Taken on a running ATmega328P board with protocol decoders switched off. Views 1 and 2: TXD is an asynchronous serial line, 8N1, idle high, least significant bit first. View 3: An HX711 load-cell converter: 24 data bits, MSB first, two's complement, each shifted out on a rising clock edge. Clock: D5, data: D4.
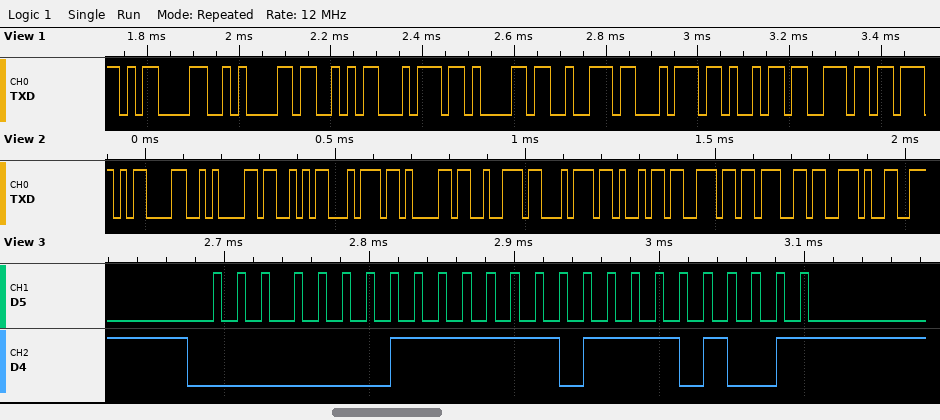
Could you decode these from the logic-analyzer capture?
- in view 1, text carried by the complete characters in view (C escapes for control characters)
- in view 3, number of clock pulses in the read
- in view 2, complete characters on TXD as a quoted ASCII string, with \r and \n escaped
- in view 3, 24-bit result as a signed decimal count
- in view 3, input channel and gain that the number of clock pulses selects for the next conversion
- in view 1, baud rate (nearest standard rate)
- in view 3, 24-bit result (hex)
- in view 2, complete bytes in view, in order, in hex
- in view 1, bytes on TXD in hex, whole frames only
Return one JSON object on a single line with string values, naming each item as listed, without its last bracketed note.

{"in view 1, text carried by the complete characters in view": "\"\\r\\nStartin\"", "in view 3, number of clock pulses in the read": "25", "in view 2, complete characters on TXD as a quoted ASCII string, with \\r and \\n escaped": "\"\\r\\nStarting.\"", "in view 3, 24-bit result as a signed decimal count": "130537", "in view 3, input channel and gain that the number of clock pulses selects for the next conversion": "channel A, gain 128", "in view 1, baud rate": "57600 baud", "in view 3, 24-bit result": "0x01FDE9", "in view 2, complete bytes in view, in order, in hex": "0D 0A 53 74 61 72 74 69 6E 67 2E", "in view 1, bytes on TXD in hex, whole frames only": "0D 0A 53 74 61 72 74 69 6E"}
